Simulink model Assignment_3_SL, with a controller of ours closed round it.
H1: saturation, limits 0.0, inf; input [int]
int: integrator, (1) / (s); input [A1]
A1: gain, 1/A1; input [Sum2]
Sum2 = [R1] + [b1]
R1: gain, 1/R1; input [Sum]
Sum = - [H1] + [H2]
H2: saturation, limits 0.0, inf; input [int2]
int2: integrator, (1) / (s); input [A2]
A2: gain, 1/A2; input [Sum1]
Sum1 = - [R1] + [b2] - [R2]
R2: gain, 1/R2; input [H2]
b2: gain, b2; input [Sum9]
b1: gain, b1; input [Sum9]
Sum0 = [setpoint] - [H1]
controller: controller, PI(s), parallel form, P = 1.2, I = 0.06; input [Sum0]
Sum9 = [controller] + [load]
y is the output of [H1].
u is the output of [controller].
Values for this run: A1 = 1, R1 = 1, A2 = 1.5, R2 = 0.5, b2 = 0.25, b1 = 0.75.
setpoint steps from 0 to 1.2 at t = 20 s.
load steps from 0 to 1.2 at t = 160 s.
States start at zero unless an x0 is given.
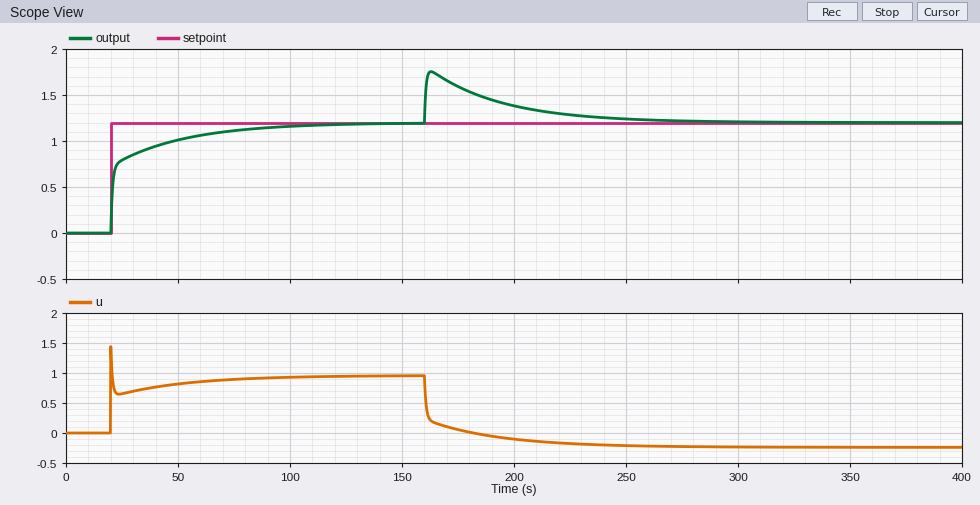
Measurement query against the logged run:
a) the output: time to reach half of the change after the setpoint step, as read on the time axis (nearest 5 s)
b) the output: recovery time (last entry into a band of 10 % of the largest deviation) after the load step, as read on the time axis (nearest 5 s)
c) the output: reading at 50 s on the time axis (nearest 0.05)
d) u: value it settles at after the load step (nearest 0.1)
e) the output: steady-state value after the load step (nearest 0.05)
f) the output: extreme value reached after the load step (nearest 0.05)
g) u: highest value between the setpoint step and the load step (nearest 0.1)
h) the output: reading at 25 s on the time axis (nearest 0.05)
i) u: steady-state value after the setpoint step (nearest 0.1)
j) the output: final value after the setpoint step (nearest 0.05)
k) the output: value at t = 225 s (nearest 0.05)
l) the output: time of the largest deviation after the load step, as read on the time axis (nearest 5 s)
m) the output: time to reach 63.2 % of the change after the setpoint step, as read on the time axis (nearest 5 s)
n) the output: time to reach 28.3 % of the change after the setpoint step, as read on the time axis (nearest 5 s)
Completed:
20 s
240 s
1.00
-0.2
1.20
1.75
1.4
0.80
1.0
1.20
1.30
165 s
25 s
20 s
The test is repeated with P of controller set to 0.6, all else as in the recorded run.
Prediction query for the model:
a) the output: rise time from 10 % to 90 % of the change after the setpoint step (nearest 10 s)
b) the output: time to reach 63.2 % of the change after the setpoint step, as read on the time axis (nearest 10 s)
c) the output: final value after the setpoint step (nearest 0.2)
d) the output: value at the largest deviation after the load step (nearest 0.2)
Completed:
40 s
30 s
1.2
2.0
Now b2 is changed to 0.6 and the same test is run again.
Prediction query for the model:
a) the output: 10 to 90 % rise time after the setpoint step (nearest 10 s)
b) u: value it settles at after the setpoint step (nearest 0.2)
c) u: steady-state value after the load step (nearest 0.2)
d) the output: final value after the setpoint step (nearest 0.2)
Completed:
40 s
0.8
-0.4
1.2
